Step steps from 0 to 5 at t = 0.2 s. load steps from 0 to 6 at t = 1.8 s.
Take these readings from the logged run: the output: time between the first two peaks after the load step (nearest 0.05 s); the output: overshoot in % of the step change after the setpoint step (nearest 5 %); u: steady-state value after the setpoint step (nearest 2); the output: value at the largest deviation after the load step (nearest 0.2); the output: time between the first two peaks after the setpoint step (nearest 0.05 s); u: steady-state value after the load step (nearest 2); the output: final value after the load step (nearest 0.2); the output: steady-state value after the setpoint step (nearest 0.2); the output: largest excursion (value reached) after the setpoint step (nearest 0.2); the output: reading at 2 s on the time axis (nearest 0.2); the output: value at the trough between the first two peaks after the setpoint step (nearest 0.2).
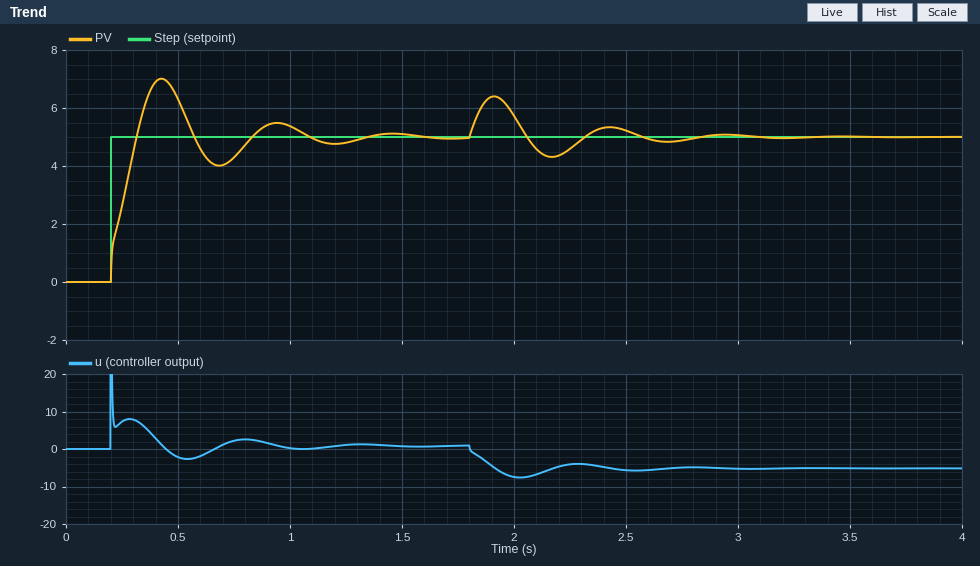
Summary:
0.50 s
40 %
0
6.4
0.50 s
-6
5.0
5.0
7.0
5.8
4.0
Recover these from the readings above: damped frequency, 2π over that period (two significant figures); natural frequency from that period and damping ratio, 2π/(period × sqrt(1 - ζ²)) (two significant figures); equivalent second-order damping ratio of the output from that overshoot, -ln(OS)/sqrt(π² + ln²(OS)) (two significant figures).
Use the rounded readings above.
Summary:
13 rad/s
13 rad/s
0.28
